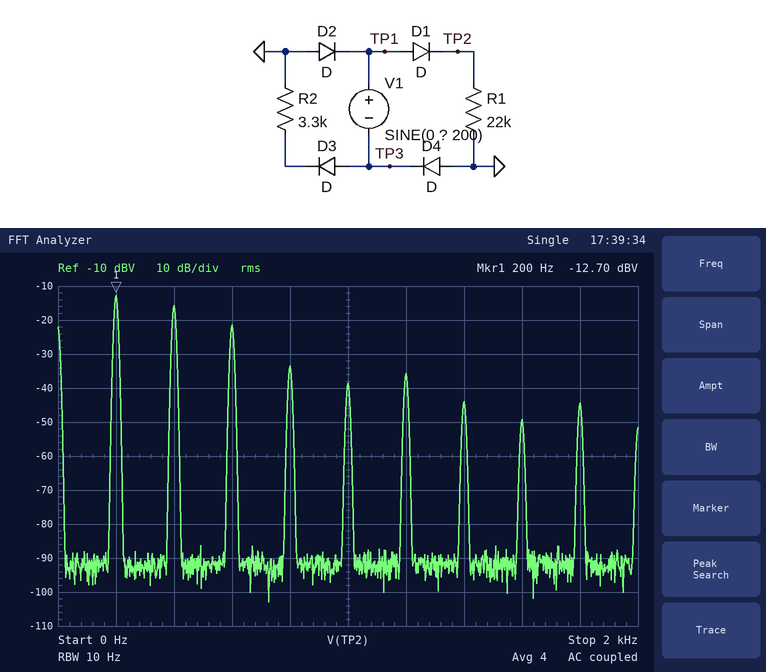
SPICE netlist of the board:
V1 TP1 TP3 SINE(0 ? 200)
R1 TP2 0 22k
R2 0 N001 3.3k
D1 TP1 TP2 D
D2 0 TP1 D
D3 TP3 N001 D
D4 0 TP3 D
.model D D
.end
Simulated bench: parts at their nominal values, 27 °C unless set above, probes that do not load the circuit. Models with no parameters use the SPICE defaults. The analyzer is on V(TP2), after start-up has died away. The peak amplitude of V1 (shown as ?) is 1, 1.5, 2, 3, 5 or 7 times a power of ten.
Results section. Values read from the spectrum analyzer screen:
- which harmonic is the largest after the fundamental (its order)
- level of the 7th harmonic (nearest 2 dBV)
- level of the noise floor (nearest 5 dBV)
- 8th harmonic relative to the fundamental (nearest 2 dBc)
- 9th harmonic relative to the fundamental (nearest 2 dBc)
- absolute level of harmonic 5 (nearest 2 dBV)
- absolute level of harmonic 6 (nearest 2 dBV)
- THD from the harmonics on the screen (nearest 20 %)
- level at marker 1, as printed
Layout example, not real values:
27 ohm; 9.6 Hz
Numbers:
2; -44 dBV; -90 dBV; -36 dBc; -32 dBc; -38 dBV; -36 dBV; 80 %; -12.70 dBV
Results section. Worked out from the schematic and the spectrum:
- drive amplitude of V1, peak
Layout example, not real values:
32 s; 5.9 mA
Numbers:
2 V
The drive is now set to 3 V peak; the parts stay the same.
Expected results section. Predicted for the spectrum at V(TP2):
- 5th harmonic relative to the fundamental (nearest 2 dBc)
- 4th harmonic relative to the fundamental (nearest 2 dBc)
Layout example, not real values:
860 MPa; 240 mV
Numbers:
-22 dBc; -32 dBc
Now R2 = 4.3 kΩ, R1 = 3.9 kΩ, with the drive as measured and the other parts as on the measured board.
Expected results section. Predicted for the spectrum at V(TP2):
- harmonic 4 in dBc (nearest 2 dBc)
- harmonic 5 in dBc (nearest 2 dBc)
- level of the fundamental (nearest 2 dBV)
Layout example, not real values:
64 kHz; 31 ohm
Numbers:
-18 dBc; -30 dBc; -14 dBV
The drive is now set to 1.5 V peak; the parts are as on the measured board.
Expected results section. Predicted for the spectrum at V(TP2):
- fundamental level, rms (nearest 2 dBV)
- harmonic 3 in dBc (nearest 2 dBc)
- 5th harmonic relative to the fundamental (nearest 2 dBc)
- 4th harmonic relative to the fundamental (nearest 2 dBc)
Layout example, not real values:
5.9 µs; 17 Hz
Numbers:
-20 dBV; -6 dBc; -24 dBc; -12 dBc
